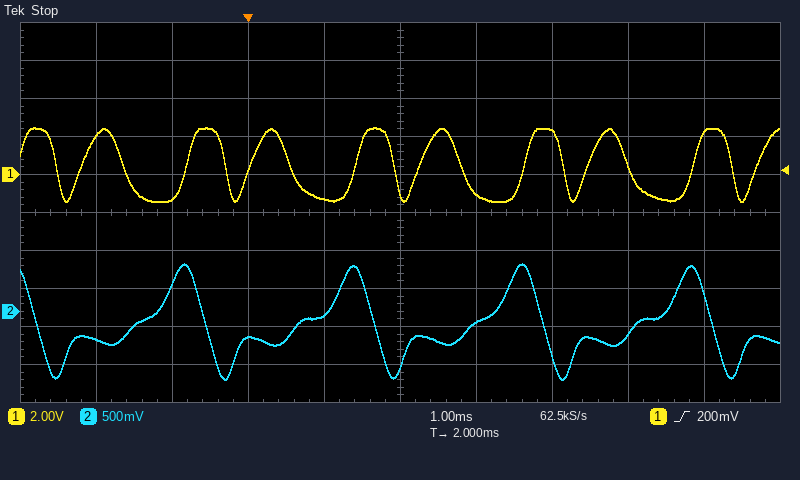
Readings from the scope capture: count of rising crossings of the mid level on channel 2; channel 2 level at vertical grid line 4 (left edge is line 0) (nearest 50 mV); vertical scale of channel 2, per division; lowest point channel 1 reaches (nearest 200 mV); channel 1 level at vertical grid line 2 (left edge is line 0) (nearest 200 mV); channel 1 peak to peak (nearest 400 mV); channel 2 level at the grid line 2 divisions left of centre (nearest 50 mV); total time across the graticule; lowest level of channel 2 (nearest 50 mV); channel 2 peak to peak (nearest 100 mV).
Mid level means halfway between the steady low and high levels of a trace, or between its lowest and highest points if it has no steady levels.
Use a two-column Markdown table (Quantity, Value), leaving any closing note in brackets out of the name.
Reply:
| Quantity | Value |
|---|---|
| count of rising crossings of the mid level on channel 2 | 4 |
| channel 2 level at vertical grid line 4 (left edge is line 0) | -50 mV |
| vertical scale of channel 2, per division | 500 mV |
| lowest point channel 1 reaches | -1.4 V |
| channel 1 level at vertical grid line 2 (left edge is line 0) | -1.2 V |
| channel 1 peak to peak | 4.0 V |
| channel 2 level at the grid line 2 divisions left of centre | -350 mV |
| total time across the graticule | 10 ms |
| lowest level of channel 2 | -900 mV |
| channel 2 peak to peak | 1.50 V |
